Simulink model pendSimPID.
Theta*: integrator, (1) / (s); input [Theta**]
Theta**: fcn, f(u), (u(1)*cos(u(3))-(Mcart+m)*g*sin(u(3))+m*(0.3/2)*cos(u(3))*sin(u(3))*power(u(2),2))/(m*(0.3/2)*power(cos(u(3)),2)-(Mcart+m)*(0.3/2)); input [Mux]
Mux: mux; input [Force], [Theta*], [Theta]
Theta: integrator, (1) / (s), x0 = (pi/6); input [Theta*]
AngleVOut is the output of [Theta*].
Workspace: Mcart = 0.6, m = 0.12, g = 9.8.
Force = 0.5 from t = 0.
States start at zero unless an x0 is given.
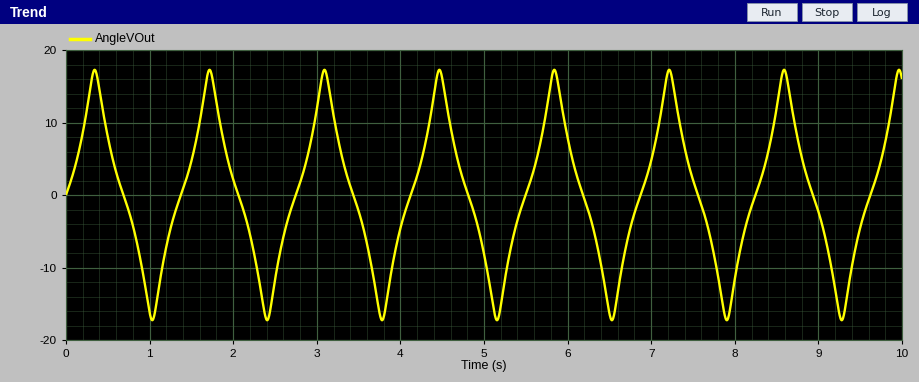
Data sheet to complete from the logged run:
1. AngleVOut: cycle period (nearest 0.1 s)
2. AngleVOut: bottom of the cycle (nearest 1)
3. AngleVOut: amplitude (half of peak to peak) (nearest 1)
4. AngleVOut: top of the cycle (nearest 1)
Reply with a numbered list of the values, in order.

1. 1.4 s
2. -17
3. 17
4. 17
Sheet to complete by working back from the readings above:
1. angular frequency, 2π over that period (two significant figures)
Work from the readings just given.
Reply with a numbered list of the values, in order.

1. 4.5 rad/s
